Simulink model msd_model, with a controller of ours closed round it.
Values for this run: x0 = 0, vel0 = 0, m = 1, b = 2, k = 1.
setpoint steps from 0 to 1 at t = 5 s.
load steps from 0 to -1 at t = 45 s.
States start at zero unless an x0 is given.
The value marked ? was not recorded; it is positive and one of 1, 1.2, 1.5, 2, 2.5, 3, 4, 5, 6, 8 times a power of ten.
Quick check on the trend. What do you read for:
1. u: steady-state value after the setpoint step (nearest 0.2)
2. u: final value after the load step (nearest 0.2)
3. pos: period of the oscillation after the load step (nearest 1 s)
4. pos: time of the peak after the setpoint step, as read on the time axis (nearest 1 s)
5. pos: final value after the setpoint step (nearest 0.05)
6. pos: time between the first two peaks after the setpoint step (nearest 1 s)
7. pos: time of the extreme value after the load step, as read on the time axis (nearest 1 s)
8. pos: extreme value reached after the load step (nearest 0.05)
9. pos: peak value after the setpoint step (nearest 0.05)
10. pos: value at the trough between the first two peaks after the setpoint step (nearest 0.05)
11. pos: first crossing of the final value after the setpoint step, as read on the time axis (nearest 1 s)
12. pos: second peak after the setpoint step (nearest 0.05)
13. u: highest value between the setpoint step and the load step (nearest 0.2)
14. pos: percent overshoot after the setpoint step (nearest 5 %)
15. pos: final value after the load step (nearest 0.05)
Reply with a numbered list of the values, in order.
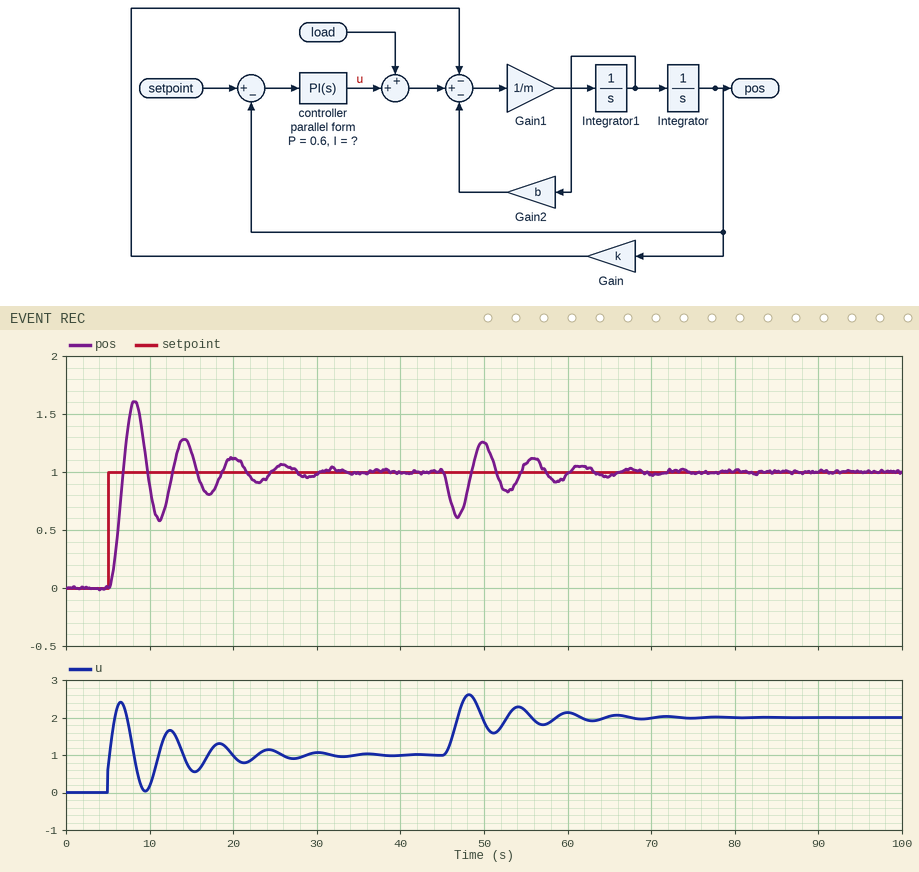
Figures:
1. 1.0
2. 2.0
3. 6 s
4. 8 s
5. 1.00
6. 6 s
7. 47 s
8. 0.60
9. 1.60
10. 0.60
11. 7 s
12. 1.30
13. 2.4
14. 60 %
15. 1.00
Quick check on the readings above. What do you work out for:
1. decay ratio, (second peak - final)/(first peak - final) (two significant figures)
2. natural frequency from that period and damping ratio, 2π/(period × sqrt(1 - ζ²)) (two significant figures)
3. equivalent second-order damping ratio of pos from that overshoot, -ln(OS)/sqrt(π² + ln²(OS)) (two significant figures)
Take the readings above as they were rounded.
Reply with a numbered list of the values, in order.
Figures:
1. 0.50
2. 1.1 rad/s
3. 0.16
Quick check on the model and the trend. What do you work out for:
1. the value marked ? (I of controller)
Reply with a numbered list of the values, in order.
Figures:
1. 2
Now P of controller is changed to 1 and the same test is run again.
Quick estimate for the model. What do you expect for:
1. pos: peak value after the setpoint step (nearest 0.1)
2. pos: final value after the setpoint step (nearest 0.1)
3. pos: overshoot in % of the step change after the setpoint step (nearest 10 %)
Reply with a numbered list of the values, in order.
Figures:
1. 1.5
2. 1.0
3. 50 %
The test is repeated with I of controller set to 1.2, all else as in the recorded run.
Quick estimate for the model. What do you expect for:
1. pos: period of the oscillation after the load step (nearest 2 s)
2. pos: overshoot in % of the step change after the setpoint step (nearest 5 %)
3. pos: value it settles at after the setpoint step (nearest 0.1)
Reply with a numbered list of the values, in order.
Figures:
1. 8 s
2. 35 %
3. 1.0
